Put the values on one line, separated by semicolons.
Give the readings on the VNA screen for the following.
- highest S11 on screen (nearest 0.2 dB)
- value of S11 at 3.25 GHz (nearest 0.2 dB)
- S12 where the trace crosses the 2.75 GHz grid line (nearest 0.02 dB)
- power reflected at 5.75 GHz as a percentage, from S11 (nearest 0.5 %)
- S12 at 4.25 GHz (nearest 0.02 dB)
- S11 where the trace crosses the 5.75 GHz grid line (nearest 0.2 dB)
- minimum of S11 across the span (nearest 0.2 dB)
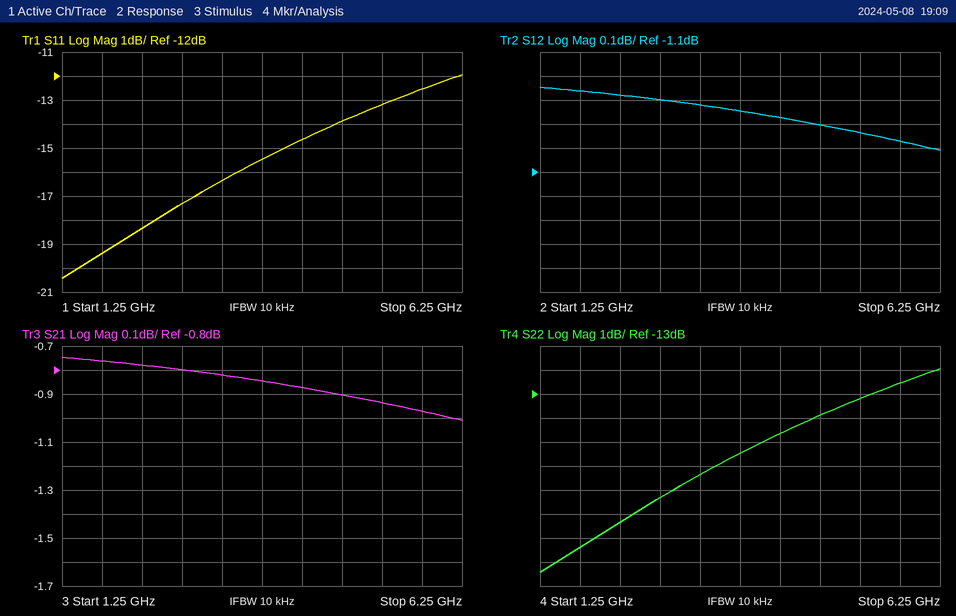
-12.0 dB; -16.4 dB; -0.80 dB; 5.5 %; -0.88 dB; -12.6 dB; -20.4 dB
